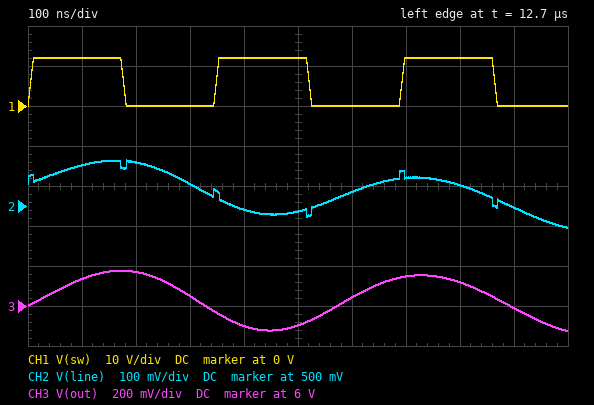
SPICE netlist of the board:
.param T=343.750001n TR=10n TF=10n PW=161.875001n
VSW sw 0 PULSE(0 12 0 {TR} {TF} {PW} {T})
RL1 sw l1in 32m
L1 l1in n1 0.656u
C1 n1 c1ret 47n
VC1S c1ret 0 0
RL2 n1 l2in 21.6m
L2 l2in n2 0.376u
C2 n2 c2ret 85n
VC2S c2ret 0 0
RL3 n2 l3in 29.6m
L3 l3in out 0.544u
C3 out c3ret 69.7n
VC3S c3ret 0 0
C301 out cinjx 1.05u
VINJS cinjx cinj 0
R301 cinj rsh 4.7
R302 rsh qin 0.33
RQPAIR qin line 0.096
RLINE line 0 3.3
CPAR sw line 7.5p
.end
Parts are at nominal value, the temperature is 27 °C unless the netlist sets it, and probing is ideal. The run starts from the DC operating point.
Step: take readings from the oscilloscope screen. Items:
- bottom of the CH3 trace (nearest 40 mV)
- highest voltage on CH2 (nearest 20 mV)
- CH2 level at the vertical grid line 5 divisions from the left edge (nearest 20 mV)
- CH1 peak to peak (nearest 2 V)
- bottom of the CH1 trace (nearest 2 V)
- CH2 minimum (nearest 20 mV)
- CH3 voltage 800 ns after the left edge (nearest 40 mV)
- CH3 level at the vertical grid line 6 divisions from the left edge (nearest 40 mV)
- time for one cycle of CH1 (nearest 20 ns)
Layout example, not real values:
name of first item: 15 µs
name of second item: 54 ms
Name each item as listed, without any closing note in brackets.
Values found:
bottom of the CH3 trace: 5.88 V
highest voltage on CH2: 620 mV
CH2 level at the vertical grid line 5 divisions from the left edge: 480 mV
CH1 peak to peak: 12 V
bottom of the CH1 trace: 0 V
CH2 minimum: 440 mV
CH3 voltage 800 ns after the left edge: 6.12 V
CH3 level at the vertical grid line 6 divisions from the left edge: 6.04 V
time for one cycle of CH1: 340 ns
